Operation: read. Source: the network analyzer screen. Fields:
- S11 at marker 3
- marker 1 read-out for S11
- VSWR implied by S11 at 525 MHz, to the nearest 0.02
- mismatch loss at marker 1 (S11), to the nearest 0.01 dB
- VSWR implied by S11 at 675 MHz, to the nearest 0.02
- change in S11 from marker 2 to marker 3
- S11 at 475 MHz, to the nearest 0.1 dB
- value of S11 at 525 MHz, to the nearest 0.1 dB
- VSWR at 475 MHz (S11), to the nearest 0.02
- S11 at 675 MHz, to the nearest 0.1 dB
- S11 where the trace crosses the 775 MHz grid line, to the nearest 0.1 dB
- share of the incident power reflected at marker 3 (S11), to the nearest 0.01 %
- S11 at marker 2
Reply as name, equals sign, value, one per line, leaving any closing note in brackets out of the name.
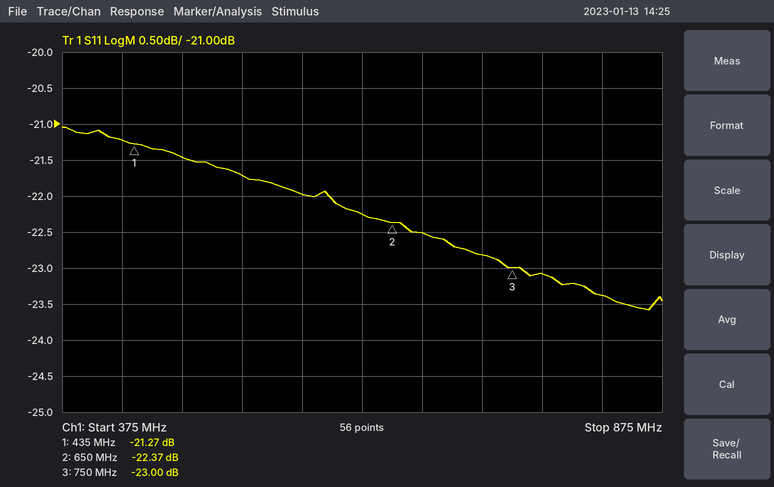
S11 at marker 3 = -23.00 dB
marker 1 read-out for S11 = -21.27 dB
VSWR implied by S11 at 525 MHz, to the nearest 0.02 = 1.18
mismatch loss at marker 1 (S11), to the nearest 0.01 dB = 0.03 dB
VSWR implied by S11 at 675 MHz, to the nearest 0.02 = 1.16
change in S11 from marker 2 to marker 3 = -0.63 dB
S11 at 475 MHz, to the nearest 0.1 dB = -21.5 dB
value of S11 at 525 MHz, to the nearest 0.1 dB = -21.7 dB
VSWR at 475 MHz (S11), to the nearest 0.02 = 1.18
S11 at 675 MHz, to the nearest 0.1 dB = -22.5 dB
S11 where the trace crosses the 775 MHz grid line, to the nearest 0.1 dB = -23.1 dB
share of the incident power reflected at marker 3 (S11), to the nearest 0.01 % = 0.50 %
S11 at marker 2 = -22.37 dB
